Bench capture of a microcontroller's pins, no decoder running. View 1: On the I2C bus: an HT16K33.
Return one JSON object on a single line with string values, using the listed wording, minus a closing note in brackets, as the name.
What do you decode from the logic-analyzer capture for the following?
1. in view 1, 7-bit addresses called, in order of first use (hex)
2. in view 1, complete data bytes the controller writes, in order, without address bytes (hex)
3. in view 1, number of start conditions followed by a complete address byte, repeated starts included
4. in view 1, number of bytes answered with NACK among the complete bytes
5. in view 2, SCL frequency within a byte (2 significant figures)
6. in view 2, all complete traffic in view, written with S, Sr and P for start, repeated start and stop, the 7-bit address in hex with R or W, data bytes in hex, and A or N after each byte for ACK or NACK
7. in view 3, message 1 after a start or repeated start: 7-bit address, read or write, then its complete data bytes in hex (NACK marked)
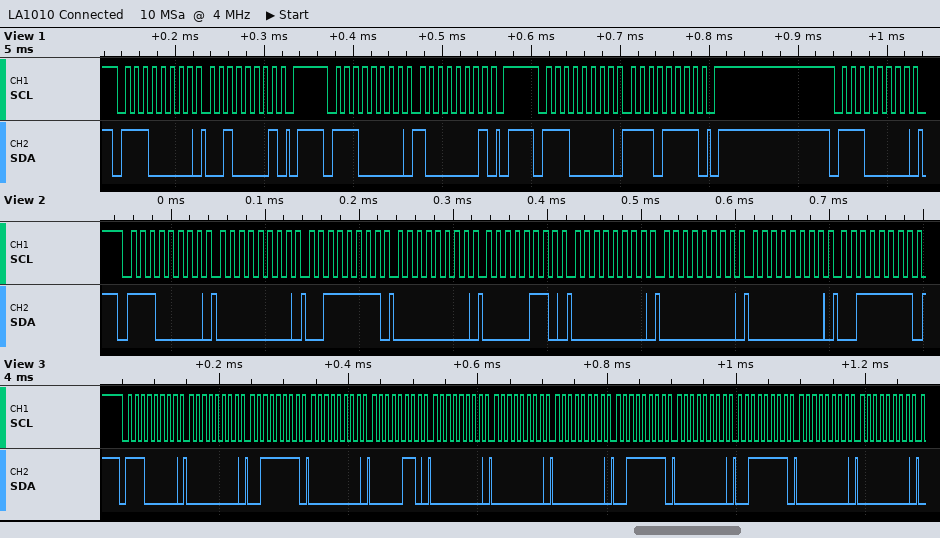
{"in view 1, 7-bit addresses called, in order of first use": "0x70", "in view 1, complete data bytes the controller writes, in order, without address bytes": "21 81 EF", "in view 1, number of start conditions followed by a complete address byte, repeated starts included": "4", "in view 1, number of bytes answered with NACK among the complete bytes": "0", "in view 2, SCL frequency within a byte": "100 kHz", "in view 2, all complete traffic in view, written with S, Sr and P for start, repeated start and stop, the 7-bit address in hex with R or W, data bytes in hex, and A or N after each byte for ACK or NACK": "S 70W A 00 A 3F A 00 A 06 A 00 A 00 A 00 A 3F A", "in view 3, message 1 after a start or repeated start: 7-bit address, read or write, then its complete data bytes in hex": "0x70 write: 00 3F 00 06 00 00 00 3F 00 3F 00 00"}
